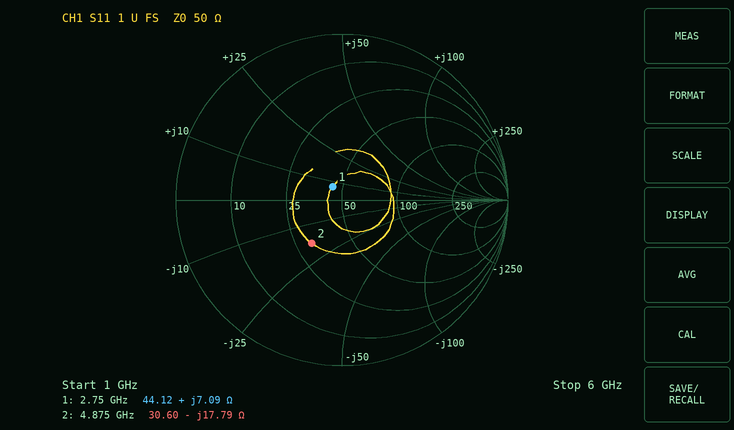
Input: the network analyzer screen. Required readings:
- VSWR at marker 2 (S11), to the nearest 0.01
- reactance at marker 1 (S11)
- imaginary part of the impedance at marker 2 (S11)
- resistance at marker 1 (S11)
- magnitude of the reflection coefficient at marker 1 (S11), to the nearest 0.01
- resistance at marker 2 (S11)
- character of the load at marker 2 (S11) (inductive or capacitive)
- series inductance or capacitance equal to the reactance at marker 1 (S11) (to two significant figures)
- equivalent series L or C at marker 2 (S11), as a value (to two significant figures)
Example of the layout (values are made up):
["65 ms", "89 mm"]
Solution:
["1.94", "+7.09 Ω", "-17.79 Ω", "44.12 Ω", "0.10", "30.60 Ω", "capacitive", "410 pH", "1.8 pF"]
